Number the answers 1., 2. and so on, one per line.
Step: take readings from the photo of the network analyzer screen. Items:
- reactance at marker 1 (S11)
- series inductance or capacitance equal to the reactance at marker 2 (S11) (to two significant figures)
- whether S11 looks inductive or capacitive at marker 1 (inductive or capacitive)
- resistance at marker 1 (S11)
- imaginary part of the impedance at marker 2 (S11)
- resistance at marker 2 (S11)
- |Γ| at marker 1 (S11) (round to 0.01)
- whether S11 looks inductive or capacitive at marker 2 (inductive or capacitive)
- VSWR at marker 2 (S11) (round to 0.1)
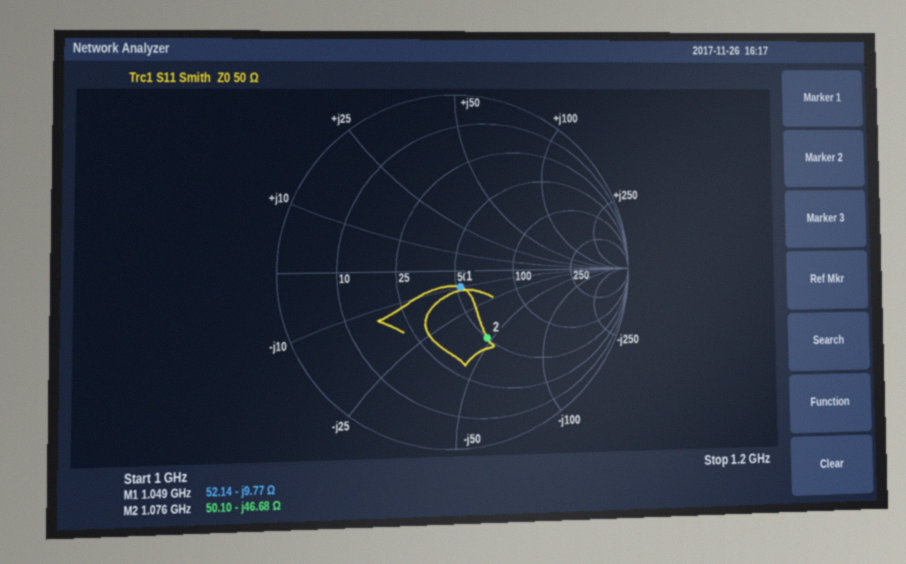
1. -9.77 Ω
2. 3.2 pF
3. capacitive
4. 52.14 Ω
5. -46.68 Ω
6. 50.10 Ω
7. 0.10
8. capacitive
9. 2.5
